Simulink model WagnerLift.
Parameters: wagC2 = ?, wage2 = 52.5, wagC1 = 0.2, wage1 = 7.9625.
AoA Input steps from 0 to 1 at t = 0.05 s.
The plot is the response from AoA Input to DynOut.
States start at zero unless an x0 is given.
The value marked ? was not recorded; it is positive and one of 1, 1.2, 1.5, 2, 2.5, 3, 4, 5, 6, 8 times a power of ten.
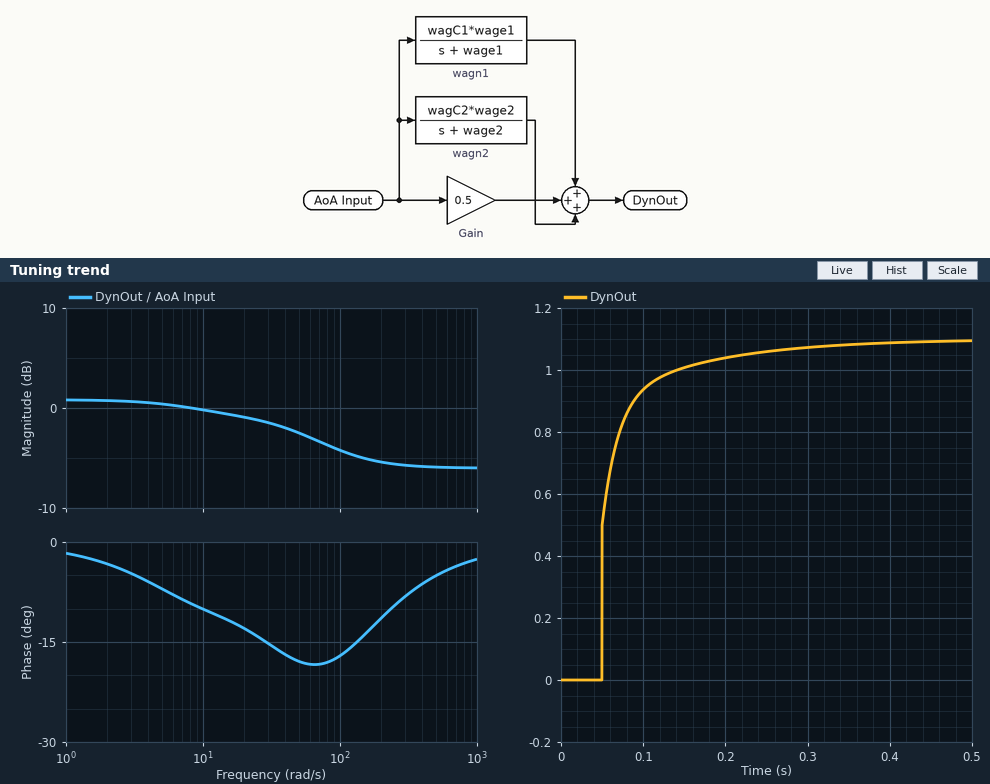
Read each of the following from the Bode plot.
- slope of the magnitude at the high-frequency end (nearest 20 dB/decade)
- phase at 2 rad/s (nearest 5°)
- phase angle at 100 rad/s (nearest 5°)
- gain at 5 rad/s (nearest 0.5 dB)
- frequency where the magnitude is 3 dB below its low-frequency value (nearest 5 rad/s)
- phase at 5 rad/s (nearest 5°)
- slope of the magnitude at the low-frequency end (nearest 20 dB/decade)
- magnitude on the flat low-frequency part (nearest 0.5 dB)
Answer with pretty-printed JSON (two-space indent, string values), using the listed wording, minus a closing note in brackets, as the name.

{
  "slope of the magnitude at the high-frequency end": "0 dB/decade",
  "phase at 2 rad/s": "-5°",
  "phase angle at 100 rad/s": "-15°",
  "gain at 5 rad/s": "0.5 dB",
  "frequency where the magnitude is 3 dB below its low-frequency value": "45 rad/s",
  "phase at 5 rad/s": "-5°",
  "slope of the magnitude at the low-frequency end": "0 dB/decade",
  "magnitude on the flat low-frequency part": "1.0 dB"
}
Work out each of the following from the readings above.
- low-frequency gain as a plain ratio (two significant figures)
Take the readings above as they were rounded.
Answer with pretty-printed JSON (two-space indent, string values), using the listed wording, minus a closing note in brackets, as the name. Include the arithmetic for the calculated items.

{
  "low-frequency gain as a plain ratio": "10^(1 / 20) = 1.1"
}
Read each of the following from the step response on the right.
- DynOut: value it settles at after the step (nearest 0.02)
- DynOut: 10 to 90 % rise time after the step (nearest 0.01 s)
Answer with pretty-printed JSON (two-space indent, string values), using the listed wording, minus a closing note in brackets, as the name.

{
  "DynOut: value it settles at after the step": "1.10",
  "DynOut: 10 to 90 % rise time after the step": "0.08 s"
}
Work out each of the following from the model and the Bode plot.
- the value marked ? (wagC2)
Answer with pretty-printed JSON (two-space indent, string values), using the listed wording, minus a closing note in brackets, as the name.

{
  "the value marked ?": "0.4"
}
